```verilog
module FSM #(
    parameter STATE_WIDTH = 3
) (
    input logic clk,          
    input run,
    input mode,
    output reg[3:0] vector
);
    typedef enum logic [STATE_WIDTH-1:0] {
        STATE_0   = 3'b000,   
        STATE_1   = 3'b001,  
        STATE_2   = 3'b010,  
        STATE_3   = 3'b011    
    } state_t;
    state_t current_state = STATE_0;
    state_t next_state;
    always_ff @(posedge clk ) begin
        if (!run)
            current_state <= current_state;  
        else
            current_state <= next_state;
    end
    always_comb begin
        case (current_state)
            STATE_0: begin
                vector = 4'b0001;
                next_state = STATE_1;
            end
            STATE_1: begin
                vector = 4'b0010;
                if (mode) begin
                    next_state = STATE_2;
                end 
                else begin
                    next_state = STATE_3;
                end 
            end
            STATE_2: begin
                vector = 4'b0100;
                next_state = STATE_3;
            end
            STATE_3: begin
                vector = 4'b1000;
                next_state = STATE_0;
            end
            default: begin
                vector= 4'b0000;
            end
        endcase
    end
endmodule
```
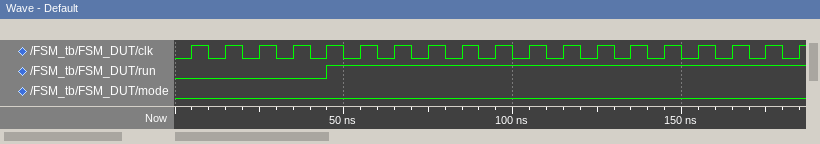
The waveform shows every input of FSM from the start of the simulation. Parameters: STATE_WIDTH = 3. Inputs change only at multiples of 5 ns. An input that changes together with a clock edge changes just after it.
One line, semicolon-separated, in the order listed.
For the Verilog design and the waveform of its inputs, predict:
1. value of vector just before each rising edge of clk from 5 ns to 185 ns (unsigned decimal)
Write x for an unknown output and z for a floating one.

1, 1, 1, 1, 1, 1, 2, 8, 1, 2, 8, 1, 2, 8, 1, 2, 8, 1, 2
